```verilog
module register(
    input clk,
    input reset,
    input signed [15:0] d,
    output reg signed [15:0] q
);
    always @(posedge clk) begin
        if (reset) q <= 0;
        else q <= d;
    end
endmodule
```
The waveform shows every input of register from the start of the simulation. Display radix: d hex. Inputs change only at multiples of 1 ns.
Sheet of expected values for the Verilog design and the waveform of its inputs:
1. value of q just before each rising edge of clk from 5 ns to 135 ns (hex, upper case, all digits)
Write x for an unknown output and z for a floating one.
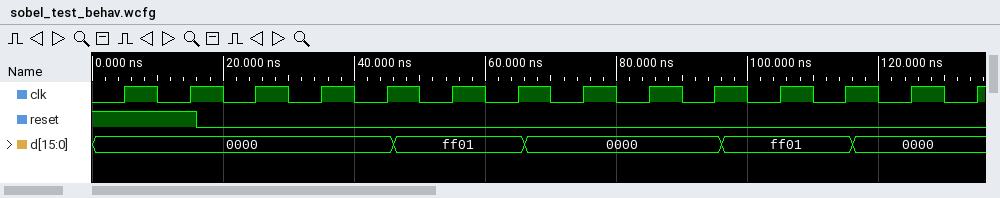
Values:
x, 0000, 0000, 0000, 0000, 0000, FF01, FF01, 0000, 0000, 0000, FF01, FF01, 0000
